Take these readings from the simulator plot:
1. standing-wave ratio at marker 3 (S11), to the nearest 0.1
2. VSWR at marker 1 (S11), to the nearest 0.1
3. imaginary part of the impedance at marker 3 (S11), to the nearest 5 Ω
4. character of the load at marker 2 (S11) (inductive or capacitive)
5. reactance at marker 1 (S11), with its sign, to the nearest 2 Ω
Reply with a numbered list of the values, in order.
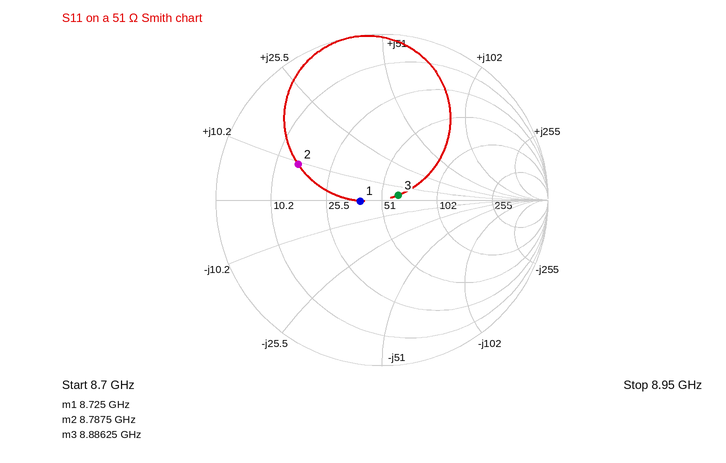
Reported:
1. 1.2
2. 1.3
3. +5 Ω
4. inductive
5. 0 Ω
